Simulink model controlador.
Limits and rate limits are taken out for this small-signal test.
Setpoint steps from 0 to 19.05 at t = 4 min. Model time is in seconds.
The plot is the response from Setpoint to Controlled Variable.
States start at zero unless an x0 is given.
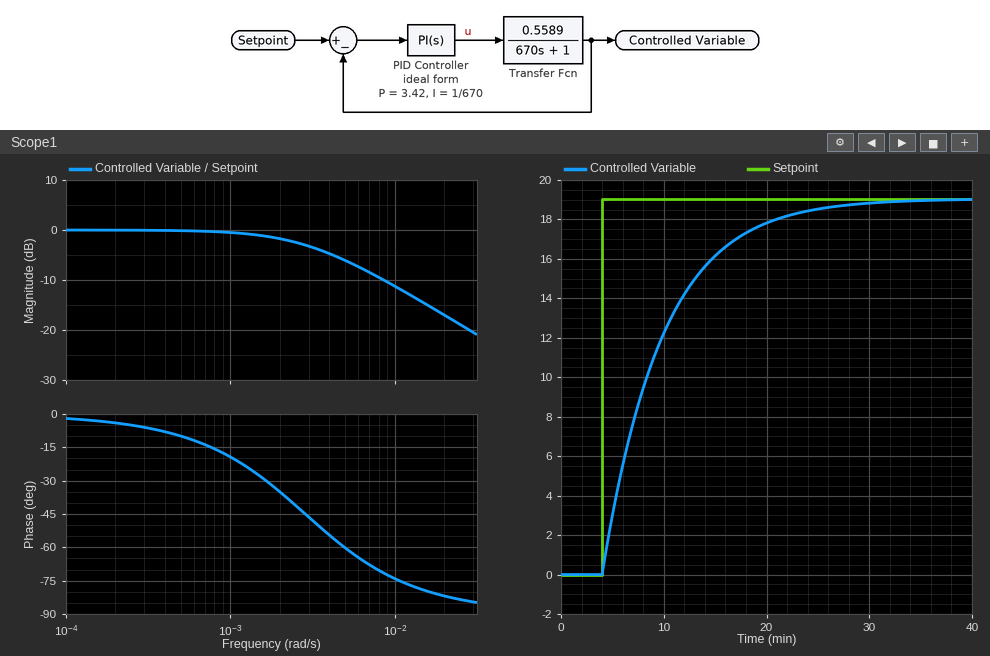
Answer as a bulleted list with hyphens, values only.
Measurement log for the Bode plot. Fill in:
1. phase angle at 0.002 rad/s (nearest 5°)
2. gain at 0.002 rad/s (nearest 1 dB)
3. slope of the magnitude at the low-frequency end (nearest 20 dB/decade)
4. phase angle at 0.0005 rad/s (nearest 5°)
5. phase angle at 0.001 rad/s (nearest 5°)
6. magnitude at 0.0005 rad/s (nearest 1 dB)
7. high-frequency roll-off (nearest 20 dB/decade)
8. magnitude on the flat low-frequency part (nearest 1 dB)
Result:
- -35°
- -2 dB
- 0 dB/decade
- -10°
- -20°
- 0 dB
- -20 dB/decade
- 0 dB
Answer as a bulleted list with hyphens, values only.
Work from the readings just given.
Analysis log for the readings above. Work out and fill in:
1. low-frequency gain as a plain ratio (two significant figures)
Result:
- 1.0
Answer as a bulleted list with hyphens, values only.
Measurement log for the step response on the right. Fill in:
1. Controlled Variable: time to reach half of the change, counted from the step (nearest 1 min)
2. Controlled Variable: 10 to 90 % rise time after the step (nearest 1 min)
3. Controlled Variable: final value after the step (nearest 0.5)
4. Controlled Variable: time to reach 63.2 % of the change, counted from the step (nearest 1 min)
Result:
- 4 min
- 13 min
- 19.0
- 6 min
